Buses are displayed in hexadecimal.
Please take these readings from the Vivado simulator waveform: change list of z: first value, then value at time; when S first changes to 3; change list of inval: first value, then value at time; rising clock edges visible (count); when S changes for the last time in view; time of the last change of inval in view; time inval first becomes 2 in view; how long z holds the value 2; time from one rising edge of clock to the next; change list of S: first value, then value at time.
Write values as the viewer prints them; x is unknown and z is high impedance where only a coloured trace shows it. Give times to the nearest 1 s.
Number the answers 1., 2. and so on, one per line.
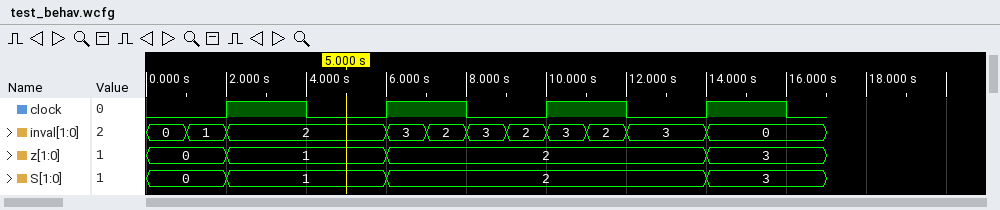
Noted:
1. 0, 1 at 2 s, 2 at 6 s, 3 at 14 s
2. 14 s
3. 0, 1 at 1 s, 2 at 2 s, 3 at 6 s, 2 at 7 s, 3 at 8 s, 2 at 9 s, 3 at 10 s, 2 at 11 s, 3 at 12 s, 0 at 14 s
4. 4
5. 14 s
6. 14 s
7. 2 s
8. 8 s
9. 4 s
10. 0, 1 at 2 s, 2 at 6 s, 3 at 14 s
